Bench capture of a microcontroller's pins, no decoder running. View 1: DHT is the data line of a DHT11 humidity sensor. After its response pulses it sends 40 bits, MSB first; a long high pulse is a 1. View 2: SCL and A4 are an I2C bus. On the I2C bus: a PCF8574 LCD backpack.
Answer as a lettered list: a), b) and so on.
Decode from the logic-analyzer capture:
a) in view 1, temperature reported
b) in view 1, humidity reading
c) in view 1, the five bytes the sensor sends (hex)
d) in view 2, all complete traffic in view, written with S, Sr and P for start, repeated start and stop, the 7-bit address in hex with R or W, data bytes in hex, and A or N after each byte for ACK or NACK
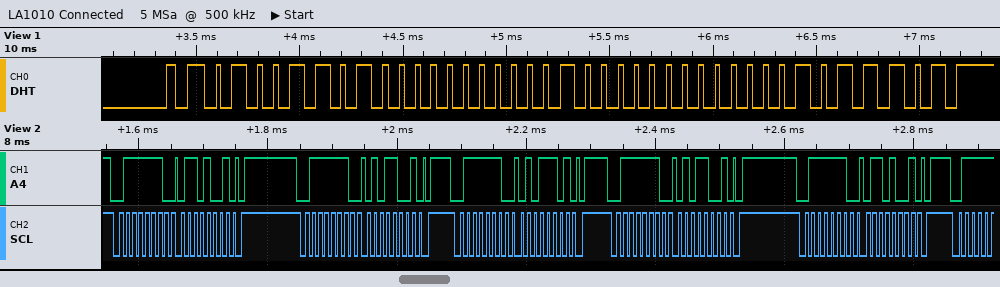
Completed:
a) 16.0 °C
b) 77 %
c) 4D 00 10 00 5D
d) S 3FW A 69 A P S 3FW A 59 A P S 3FW A 5D A P S 3FW A 59 A P S 3FW A 69 A P
